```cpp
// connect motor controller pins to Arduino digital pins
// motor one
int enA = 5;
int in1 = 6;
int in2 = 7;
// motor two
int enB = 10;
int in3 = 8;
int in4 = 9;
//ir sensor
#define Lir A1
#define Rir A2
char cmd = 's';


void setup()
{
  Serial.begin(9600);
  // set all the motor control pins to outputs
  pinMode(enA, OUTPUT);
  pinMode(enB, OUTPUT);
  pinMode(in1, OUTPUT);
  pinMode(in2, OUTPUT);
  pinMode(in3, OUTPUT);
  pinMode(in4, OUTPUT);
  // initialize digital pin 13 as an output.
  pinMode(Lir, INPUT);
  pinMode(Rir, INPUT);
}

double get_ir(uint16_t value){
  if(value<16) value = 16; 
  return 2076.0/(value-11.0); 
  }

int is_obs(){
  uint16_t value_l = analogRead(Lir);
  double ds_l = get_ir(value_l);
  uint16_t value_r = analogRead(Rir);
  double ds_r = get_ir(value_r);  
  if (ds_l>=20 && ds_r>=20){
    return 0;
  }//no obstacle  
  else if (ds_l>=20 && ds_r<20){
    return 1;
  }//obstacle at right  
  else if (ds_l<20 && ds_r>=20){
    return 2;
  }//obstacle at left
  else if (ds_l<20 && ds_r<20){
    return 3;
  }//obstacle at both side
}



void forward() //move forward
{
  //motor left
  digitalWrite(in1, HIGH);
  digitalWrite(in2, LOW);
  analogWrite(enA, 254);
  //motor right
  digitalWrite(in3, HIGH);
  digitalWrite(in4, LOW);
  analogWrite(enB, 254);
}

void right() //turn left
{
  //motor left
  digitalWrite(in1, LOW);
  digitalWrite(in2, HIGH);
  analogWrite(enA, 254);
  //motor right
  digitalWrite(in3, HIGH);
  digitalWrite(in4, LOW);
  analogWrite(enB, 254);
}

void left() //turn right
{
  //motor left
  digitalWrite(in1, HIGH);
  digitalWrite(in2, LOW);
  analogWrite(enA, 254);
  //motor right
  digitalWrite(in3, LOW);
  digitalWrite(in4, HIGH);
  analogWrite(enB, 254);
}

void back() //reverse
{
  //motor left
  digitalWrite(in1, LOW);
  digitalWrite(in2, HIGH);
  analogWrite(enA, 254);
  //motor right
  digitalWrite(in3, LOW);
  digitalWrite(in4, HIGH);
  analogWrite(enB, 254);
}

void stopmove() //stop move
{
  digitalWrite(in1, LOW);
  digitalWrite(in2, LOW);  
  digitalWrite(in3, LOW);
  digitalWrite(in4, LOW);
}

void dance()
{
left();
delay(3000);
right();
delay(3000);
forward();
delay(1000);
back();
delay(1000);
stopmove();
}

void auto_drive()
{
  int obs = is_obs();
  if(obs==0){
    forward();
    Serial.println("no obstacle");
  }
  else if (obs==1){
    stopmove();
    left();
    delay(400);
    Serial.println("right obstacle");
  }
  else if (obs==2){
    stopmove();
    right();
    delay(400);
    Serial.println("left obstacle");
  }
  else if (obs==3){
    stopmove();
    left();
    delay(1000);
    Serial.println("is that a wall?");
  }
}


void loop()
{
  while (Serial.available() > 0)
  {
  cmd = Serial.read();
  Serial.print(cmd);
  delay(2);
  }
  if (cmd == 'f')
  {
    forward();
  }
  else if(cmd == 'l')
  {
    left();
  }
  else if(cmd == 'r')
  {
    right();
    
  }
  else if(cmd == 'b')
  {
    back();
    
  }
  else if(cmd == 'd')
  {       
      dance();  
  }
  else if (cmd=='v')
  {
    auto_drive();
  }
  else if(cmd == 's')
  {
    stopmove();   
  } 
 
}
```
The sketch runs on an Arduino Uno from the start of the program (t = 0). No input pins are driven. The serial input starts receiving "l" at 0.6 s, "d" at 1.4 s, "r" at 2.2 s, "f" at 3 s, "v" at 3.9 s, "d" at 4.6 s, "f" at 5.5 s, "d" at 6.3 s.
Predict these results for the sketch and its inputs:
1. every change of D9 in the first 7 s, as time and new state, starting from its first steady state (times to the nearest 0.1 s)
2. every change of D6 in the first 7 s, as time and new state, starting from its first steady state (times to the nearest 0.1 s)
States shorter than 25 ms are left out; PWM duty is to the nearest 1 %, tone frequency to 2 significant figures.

0 s low; 0.6 s high; 4.4 s low
0 s low; 0.6 s high; 4.4 s low
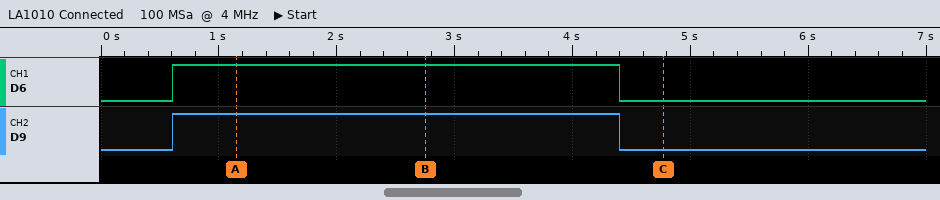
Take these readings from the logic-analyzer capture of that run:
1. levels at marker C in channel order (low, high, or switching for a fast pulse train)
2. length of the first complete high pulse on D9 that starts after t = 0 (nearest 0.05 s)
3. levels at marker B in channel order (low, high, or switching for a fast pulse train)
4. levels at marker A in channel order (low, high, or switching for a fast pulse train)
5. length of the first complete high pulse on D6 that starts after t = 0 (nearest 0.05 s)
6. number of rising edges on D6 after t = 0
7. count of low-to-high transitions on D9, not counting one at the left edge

D6 low, D9 low
3.80 s
D6 high, D9 high
D6 high, D9 high
3.80 s
1
1
